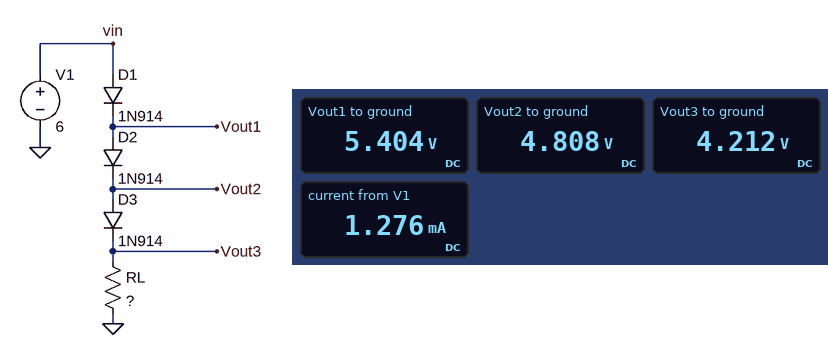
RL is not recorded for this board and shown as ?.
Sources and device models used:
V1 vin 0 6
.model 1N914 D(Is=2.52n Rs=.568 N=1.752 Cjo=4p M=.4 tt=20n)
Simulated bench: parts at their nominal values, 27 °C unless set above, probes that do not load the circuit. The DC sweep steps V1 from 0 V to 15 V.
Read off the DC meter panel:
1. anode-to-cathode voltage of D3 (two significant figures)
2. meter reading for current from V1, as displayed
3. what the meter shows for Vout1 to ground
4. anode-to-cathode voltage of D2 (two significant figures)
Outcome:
600 mV
1.276 mA
5.404 V
600 mV
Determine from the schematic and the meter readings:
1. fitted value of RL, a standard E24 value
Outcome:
3.3 kΩ
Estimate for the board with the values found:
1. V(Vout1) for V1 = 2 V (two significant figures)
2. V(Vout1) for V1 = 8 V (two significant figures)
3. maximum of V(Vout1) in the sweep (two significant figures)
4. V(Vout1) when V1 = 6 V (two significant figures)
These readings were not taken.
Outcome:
1.5 V
7.4 V
14 V
5.4 V
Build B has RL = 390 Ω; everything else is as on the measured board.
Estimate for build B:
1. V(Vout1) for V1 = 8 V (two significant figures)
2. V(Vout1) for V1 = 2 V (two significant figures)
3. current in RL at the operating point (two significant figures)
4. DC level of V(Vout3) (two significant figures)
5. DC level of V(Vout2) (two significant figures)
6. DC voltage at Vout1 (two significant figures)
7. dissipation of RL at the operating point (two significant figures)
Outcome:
7.3 V
1.4 V
10 mA
3.9 V
4.6 V
5.3 V
39 mW
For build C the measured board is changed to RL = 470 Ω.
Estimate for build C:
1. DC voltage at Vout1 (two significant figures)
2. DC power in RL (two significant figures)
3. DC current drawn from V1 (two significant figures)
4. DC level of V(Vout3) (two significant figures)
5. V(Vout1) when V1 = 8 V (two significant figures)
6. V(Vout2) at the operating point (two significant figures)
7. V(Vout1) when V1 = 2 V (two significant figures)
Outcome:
5.3 V
33 mW
8.4 mA
3.9 V
7.3 V
4.6 V
1.4 V
